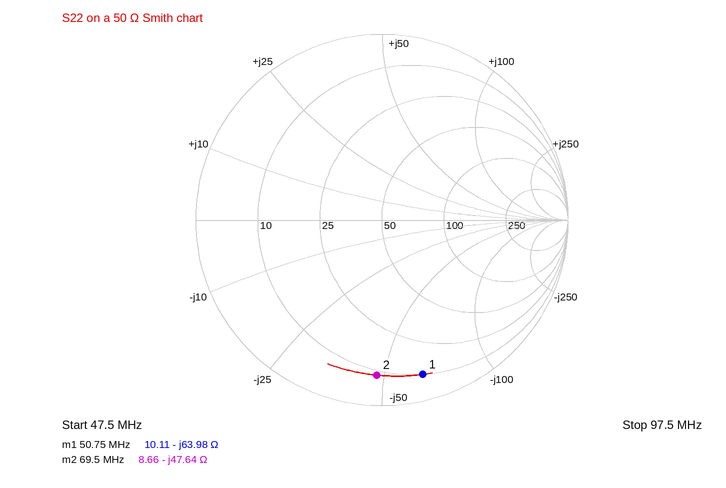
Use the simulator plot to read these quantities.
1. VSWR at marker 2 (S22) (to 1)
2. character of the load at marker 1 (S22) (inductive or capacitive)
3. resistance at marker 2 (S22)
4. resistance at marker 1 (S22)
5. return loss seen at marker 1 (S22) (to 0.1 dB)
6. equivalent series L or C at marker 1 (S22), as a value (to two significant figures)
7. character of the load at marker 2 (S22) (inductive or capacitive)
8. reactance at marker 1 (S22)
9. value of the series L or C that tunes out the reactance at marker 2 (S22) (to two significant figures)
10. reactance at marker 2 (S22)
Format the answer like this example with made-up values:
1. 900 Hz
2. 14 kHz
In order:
1. 11
2. capacitive
3. 8.66 Ω
4. 10.11 Ω
5. 1.3 dB
6. 49 pF
7. capacitive
8. -63.98 Ω
9. 110 nH
10. -47.64 Ω
